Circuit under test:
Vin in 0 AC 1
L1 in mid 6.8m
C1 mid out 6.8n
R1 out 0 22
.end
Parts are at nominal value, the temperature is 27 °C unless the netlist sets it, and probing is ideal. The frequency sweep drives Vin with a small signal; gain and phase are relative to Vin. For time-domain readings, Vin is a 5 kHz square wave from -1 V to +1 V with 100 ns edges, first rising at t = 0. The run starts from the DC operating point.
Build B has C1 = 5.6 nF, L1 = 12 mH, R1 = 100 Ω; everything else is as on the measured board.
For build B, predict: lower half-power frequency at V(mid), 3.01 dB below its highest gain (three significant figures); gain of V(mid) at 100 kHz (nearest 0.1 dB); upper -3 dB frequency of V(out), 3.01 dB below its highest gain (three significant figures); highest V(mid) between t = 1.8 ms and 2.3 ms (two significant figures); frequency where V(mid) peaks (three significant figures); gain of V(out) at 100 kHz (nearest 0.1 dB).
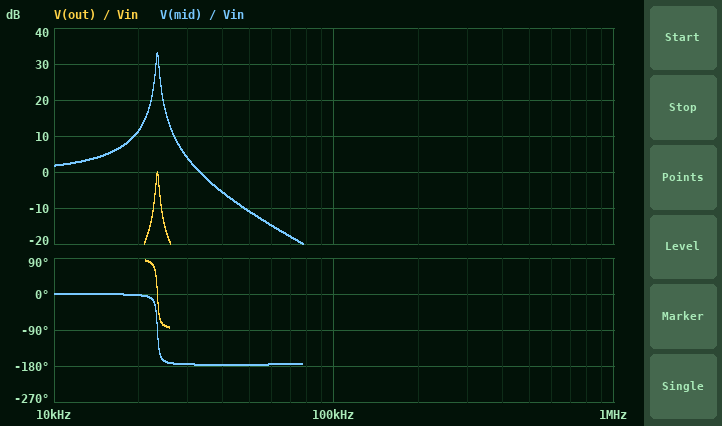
18.7 kHz
-27.6 dB
20.1 kHz
2.1 V
19.4 kHz
-37.2 dB
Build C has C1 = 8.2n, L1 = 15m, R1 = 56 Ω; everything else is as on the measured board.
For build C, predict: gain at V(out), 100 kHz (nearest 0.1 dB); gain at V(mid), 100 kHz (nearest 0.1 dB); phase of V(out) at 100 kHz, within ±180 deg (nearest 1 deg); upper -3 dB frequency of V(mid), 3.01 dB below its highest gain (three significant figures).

-44.3 dB
-33.2 dB
-90 deg
14.6 kHz
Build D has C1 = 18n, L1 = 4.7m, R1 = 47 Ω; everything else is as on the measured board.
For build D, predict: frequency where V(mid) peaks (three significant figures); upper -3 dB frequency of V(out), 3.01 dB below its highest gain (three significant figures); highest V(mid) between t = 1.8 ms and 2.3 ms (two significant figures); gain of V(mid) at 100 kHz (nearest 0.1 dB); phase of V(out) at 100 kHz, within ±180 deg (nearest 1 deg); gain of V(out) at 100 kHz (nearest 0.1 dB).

17.3 kHz
18.1 kHz
2.6 V
-29.1 dB
-89 deg
-35.7 dB
